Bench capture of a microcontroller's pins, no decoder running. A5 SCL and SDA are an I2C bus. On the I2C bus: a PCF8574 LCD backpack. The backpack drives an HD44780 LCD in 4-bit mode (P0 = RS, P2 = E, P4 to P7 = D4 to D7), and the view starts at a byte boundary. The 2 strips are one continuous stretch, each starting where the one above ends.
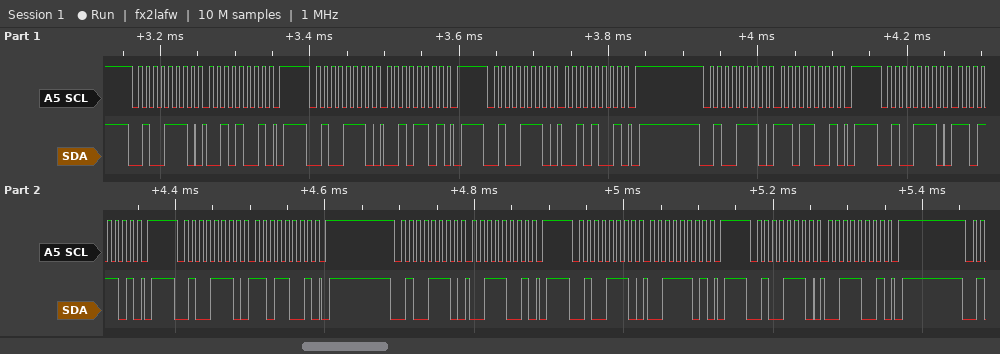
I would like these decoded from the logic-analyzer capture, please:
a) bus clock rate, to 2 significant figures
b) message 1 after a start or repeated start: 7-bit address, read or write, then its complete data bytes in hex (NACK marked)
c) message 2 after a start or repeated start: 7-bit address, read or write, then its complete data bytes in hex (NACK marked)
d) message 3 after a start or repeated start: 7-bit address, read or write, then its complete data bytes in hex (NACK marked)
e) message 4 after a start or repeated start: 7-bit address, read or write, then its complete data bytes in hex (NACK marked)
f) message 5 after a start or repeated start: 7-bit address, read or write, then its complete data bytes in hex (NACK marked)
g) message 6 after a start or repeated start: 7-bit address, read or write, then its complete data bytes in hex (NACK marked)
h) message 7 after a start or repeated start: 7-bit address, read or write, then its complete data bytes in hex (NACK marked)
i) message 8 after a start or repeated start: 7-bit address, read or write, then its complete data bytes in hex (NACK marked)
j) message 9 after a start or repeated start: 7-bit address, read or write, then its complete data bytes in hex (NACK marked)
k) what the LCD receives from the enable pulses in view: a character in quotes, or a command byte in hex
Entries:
100 kHz
0x27 write: 29
0x27 write: 2D
0x27 write: 29
0x27 write: D9
0x27 write: DD
0x27 write: D9
0x27 write: 39
0x27 write: 3D
0x27 write: 39
'-'
